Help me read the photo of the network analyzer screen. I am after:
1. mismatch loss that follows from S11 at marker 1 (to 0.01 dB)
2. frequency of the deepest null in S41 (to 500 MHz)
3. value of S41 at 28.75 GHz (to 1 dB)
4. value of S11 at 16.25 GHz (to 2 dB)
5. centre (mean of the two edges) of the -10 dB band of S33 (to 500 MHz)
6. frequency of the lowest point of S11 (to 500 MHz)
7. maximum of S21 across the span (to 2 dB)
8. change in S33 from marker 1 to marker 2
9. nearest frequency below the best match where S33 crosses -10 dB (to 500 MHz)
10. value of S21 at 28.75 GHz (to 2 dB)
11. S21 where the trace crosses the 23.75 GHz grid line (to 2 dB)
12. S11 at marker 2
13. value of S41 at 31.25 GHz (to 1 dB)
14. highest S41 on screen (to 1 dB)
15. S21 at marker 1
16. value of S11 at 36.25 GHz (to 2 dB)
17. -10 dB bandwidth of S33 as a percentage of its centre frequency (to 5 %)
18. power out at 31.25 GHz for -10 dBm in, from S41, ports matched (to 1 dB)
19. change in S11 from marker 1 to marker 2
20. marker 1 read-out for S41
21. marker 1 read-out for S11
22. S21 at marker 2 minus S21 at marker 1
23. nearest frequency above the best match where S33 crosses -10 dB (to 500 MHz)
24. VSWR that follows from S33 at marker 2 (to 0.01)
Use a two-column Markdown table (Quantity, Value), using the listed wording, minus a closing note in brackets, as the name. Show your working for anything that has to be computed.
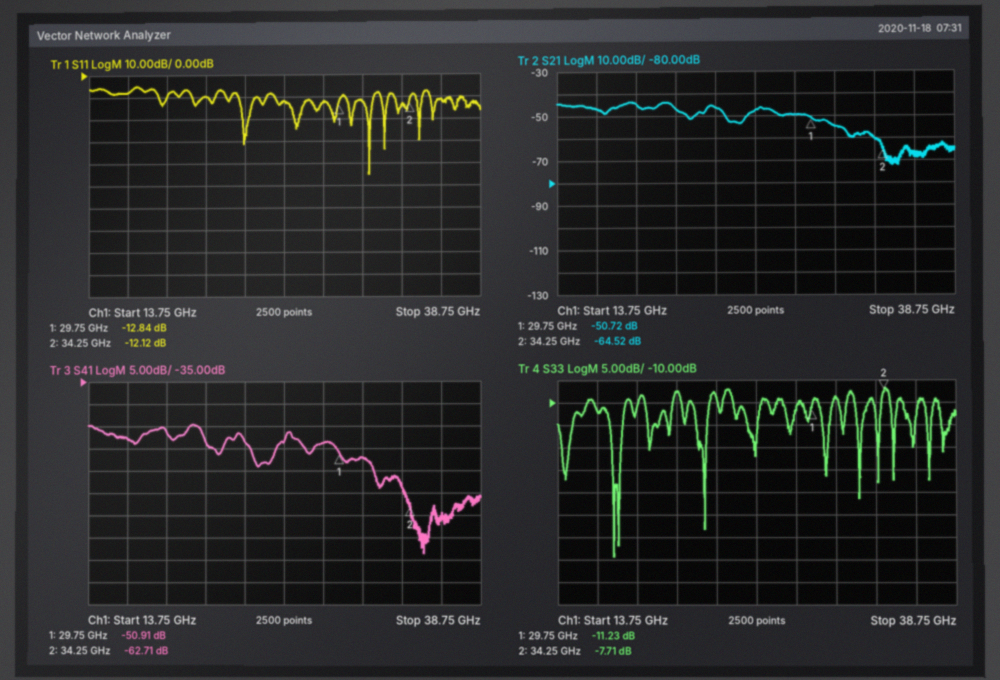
| Quantity | Value |
|---|---|
| mismatch loss that follows from S11 at marker 1 | −10 log10(1 − 10^(-12.84/10)) ≈ 0.23 dB |
| frequency of the deepest null in S41 | 35.0 GHz |
| value of S41 at 28.75 GHz | -49 dB |
| value of S11 at 16.25 GHz | -8 dB |
| centre (mean of the two edges) of the -10 dB band of S33 | 17.0 GHz |
| frequency of the lowest point of S11 | 31.5 GHz |
| maximum of S21 across the span | -44 dB |
| change in S33 from marker 1 to marker 2 | -7.71 − (-11.23) = 3.52 dB |
| nearest frequency below the best match where S33 crosses -10 dB | 16.0 GHz |
| value of S21 at 28.75 GHz | -50 dB |
| S21 where the trace crosses the 23.75 GHz grid line | -46 dB |
| S11 at marker 2 | -12.12 dB |
| value of S41 at 31.25 GHz | -52 dB |
| highest S41 on screen | -45 dB |
| S21 at marker 1 | -50.72 dB |
| value of S11 at 36.25 GHz | -12 dB |
| -10 dB bandwidth of S33 as a percentage of its centre frequency | 2 GHz / 17 GHz ≈ 11.8 %, so 10 % to the nearest 5 % |
| power out at 31.25 GHz for -10 dBm in, from S41, ports matched | -10 dBm + (-52 dB) = -62 dBm |
| change in S11 from marker 1 to marker 2 | -12.12 − (-12.84) = 0.72 dB |
| marker 1 read-out for S41 | -50.91 dB |
| marker 1 read-out for S11 | -12.84 dB |
| S21 at marker 2 minus S21 at marker 1 | -64.52 − (-50.72) = -13.80 dB |
| nearest frequency above the best match where S33 crosses -10 dB | 18.0 GHz |
| VSWR that follows from S33 at marker 2 | (1 + 0.4116)/(1 − 0.4116) ≈ 2.40 |
